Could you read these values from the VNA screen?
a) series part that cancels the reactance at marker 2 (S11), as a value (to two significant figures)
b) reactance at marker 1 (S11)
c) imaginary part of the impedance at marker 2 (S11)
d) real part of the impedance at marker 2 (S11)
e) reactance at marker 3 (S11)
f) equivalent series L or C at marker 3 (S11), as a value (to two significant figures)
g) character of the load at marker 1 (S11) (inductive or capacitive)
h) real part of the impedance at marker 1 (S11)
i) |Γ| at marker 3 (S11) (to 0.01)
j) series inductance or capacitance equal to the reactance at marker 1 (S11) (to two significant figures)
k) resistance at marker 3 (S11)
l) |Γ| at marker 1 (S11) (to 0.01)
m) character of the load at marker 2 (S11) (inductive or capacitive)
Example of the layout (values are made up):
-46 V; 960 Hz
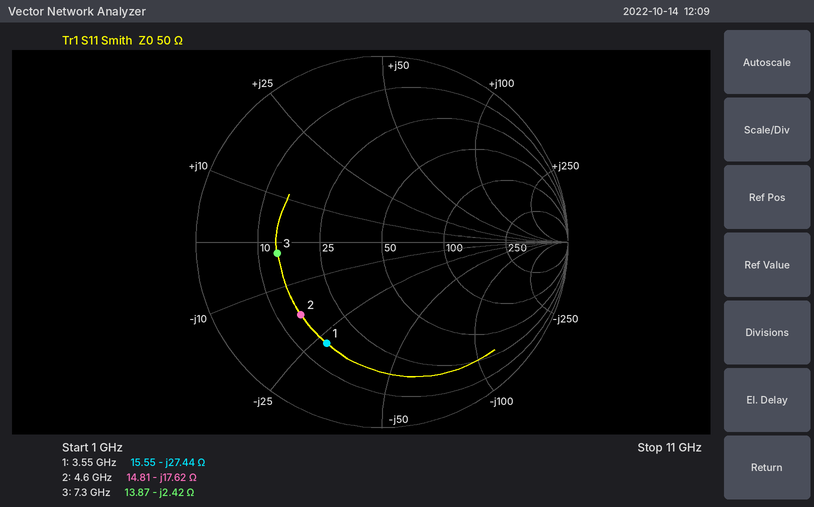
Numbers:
610 pH; -27.44 Ω; -17.62 Ω; 14.81 Ω; -2.42 Ω; 9.0 pF; capacitive; 15.55 Ω; 0.57; 1.6 pF; 13.87 Ω; 0.62; capacitive
